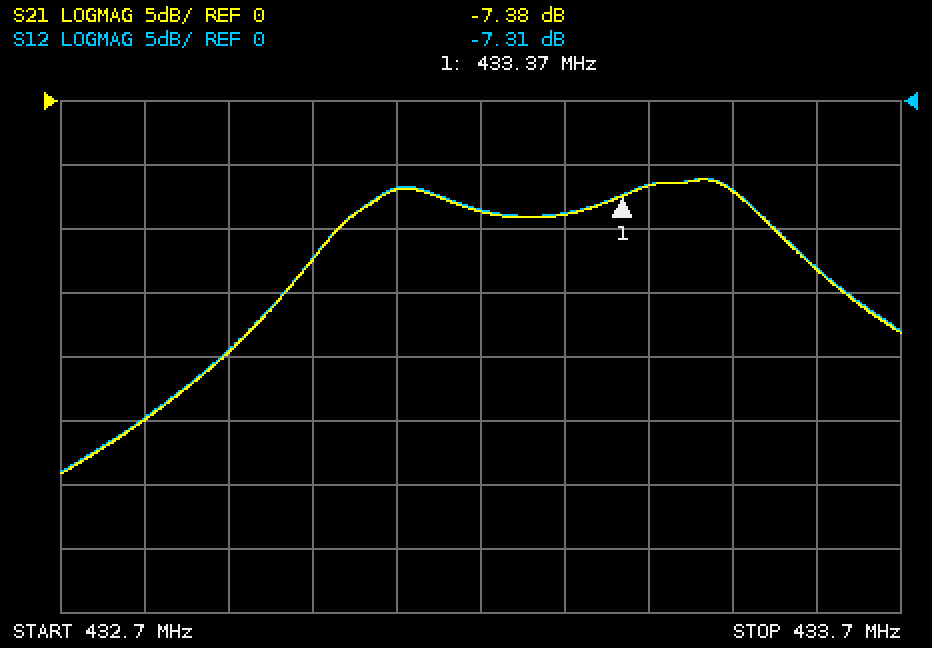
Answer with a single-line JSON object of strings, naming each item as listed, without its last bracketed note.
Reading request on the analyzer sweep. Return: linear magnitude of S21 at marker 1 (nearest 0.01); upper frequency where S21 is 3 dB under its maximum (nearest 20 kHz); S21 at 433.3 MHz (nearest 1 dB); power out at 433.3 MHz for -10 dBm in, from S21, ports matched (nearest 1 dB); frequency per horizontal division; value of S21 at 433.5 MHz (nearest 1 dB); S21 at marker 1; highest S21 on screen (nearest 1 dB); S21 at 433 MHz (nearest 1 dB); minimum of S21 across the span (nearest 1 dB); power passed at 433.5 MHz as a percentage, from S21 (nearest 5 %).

{"linear magnitude of S21 at marker 1": "0.43", "upper frequency where S21 is 3 dB under its maximum": "433.54 MHz", "S21 at 433.3 MHz": "-9 dB", "power out at 433.3 MHz for -10 dBm in, from S21, ports matched": "-19 dBm", "frequency per horizontal division": "100 kHz", "value of S21 at 433.5 MHz": "-7 dB", "S21 at marker 1": "-7.38 dB", "highest S21 on screen": "-6 dB", "S21 at 433 MHz": "-12 dB", "minimum of S21 across the span": "-29 dB", "power passed at 433.5 MHz as a percentage, from S21": "20 %"}
